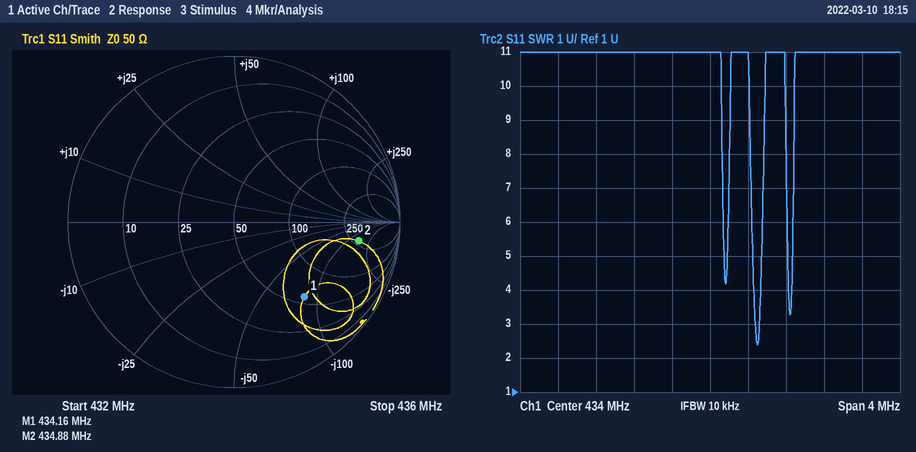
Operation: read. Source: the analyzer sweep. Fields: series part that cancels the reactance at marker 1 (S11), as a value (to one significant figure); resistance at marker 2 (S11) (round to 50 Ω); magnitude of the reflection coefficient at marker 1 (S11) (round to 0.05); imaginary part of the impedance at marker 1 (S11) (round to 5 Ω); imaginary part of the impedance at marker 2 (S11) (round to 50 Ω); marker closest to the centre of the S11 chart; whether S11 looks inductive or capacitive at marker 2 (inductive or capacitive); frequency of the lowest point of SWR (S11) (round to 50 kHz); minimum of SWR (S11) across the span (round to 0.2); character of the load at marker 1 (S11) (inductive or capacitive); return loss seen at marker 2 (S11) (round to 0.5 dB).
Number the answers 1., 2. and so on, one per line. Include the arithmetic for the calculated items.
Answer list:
1. L = 85 Ω/(2π × 434.16 MHz) ≈ 31.2 nH, so 30 nH to one significant figure
2. 300 Ω
3. 0.60
4. -85 Ω
5. -150 Ω
6. marker 1
7. capacitive
8. 434.50 MHz
9. 2.4
10. capacitive
11. 2.5 dB
